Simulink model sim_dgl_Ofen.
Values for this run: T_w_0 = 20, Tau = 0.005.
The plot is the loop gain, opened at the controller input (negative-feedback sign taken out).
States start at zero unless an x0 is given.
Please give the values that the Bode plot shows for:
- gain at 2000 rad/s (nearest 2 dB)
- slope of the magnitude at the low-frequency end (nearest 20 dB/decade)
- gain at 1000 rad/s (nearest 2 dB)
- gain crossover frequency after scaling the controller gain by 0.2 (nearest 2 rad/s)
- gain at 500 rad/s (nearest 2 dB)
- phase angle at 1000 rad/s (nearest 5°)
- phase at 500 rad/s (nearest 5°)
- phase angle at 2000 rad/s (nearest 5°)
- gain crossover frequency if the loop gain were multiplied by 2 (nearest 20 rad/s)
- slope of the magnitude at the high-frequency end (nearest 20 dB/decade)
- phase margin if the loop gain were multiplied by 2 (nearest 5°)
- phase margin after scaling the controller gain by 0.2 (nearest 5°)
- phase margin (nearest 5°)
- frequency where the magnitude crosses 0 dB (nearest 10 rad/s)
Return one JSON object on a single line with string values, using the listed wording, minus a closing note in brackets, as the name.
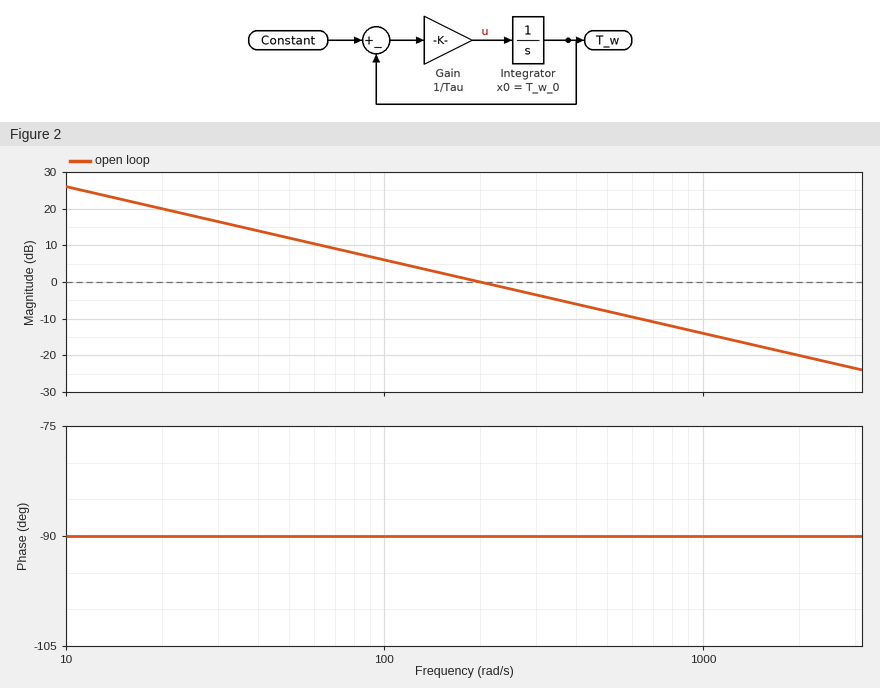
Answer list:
{"gain at 2000 rad/s": "-20 dB", "slope of the magnitude at the low-frequency end": "-20 dB/decade", "gain at 1000 rad/s": "-14 dB", "gain crossover frequency after scaling the controller gain by 0.2": "40 rad/s", "gain at 500 rad/s": "-8 dB", "phase angle at 1000 rad/s": "-90°", "phase at 500 rad/s": "-90°", "phase angle at 2000 rad/s": "-90°", "gain crossover frequency if the loop gain were multiplied by 2": "400 rad/s", "slope of the magnitude at the high-frequency end": "-20 dB/decade", "phase margin if the loop gain were multiplied by 2": "90°", "phase margin after scaling the controller gain by 0.2": "90°", "phase margin": "90°", "frequency where the magnitude crosses 0 dB": "200 rad/s"}
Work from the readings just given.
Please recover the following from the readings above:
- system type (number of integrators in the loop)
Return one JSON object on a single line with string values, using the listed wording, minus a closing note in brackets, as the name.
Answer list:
{"system type": "1"}
